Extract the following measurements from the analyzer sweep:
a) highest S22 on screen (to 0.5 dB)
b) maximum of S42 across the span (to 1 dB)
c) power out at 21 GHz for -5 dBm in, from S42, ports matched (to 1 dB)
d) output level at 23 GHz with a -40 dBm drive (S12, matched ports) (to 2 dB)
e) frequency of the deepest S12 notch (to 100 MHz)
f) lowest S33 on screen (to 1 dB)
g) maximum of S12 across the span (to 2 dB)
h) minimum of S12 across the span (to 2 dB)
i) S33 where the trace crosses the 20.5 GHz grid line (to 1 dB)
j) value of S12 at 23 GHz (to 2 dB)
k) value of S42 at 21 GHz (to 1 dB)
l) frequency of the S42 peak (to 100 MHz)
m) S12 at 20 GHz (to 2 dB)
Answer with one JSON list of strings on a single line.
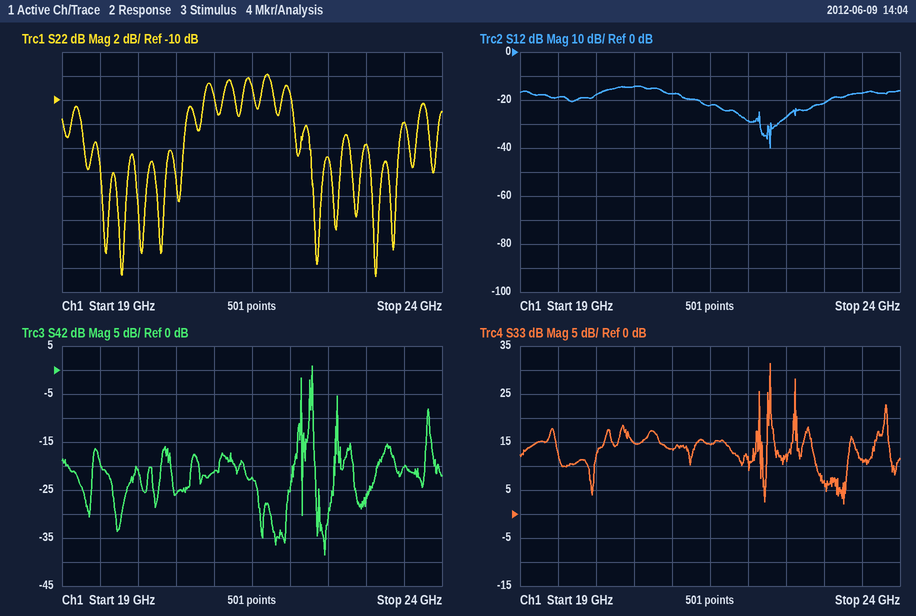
["-8.0 dB", "1 dB", "-26 dBm", "-62 dBm", "22.3 GHz", "2 dB", "-14 dB", "-40 dB", "15 dB", "-22 dB", "-21 dB", "22.3 GHz", "-18 dB"]
